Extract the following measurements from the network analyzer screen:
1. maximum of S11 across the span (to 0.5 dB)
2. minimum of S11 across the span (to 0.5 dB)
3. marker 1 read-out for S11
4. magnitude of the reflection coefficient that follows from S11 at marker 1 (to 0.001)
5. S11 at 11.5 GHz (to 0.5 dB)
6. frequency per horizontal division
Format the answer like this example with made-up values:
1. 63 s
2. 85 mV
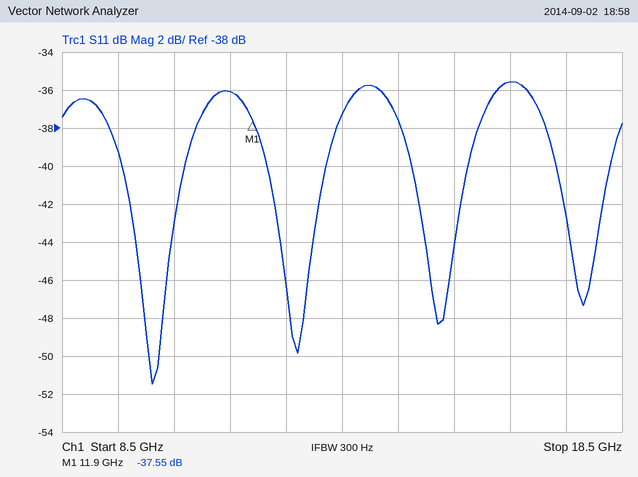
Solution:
1. -35.5 dB
2. -51.5 dB
3. -37.55 dB
4. 0.013
5. -36.0 dB
6. 1 GHz
